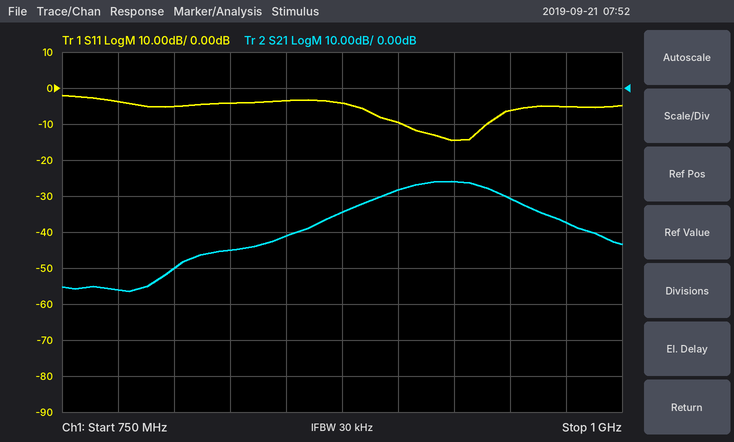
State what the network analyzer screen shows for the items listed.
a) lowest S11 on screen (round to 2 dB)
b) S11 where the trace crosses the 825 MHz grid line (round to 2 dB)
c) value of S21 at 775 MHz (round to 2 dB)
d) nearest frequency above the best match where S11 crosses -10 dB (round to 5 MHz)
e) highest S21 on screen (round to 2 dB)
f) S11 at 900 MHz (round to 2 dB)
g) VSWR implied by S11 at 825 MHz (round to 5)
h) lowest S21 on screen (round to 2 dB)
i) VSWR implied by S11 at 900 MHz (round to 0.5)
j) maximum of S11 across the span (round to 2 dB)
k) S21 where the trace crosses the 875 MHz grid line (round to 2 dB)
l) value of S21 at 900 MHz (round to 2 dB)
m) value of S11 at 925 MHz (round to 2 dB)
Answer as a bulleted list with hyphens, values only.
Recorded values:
- -14 dB
- -4 dB
- -56 dB
- 940 MHz
- -26 dB
- -10 dB
- 5
- -56 dB
- 2.0
- -2 dB
- -34 dB
- -28 dB
- -14 dB
